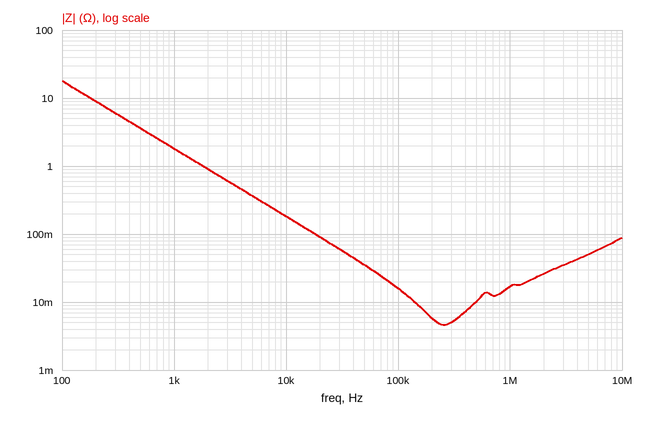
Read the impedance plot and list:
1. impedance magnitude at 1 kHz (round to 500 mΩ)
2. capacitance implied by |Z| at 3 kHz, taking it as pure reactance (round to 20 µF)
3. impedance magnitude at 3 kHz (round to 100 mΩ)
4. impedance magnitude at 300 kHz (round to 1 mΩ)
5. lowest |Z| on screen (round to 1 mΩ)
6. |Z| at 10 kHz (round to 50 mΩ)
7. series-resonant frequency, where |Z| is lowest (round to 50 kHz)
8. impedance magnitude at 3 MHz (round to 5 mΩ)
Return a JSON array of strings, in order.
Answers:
["2.0 Ω", "80 µF", "600 mΩ", "5 mΩ", "5 mΩ", "200 mΩ", "250 kHz", "35 mΩ"]
